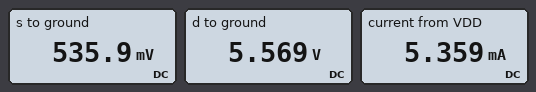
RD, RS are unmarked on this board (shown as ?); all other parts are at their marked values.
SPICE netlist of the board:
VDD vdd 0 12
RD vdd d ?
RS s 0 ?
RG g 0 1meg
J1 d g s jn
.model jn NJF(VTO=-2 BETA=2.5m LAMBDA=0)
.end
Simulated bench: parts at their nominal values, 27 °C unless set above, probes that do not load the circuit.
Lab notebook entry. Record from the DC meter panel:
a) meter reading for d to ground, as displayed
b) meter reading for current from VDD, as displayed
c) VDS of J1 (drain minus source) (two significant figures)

5.569 V
5.359 mA
5.0 V
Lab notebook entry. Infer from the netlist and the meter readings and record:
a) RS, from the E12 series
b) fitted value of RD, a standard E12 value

100 Ω
1.2 kΩ
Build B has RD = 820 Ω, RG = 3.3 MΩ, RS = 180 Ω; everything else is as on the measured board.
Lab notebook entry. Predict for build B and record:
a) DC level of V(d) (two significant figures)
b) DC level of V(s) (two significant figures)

8.7 V
730 mV
